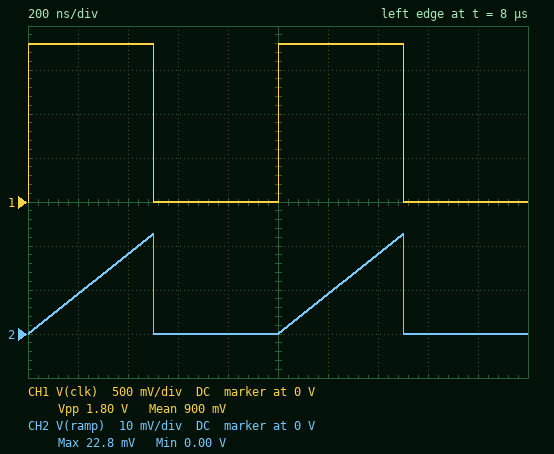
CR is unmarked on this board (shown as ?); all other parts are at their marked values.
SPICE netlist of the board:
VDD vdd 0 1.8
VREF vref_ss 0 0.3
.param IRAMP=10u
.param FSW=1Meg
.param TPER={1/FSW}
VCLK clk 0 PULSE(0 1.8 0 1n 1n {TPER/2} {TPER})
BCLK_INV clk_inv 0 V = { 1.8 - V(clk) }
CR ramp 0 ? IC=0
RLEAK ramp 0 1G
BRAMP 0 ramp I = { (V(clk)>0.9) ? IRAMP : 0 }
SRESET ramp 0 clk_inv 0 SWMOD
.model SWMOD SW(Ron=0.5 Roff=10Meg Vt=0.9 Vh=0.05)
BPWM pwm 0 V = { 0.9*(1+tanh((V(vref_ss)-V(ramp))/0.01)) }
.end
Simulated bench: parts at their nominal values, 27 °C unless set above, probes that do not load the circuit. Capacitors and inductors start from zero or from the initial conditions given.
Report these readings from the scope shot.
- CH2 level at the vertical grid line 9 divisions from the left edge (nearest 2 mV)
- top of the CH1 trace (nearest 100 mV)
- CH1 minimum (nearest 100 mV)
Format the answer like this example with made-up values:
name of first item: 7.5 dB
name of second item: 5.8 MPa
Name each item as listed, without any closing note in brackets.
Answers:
CH2 level at the vertical grid line 9 divisions from the left edge: 0 V
top of the CH1 trace: 1.8 V
CH1 minimum: 0 V
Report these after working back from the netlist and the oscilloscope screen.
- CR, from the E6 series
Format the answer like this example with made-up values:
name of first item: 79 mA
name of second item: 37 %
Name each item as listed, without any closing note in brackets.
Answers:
CR, from the E6 series: 220 pF
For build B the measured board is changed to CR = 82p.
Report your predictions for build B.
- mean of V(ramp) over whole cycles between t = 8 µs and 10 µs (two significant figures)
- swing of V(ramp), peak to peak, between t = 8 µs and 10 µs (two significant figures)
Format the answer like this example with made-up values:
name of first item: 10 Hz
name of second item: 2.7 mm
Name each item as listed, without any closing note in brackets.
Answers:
mean of V(ramp) over whole cycles between t = 8 µs and 10 µs: 15 mV
swing of V(ramp), peak to peak, between t = 8 µs and 10 µs: 61 mV
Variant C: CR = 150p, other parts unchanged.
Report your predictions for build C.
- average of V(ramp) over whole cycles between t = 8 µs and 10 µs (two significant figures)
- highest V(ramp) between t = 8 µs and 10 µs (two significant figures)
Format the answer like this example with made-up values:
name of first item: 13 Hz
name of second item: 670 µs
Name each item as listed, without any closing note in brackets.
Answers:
average of V(ramp) over whole cycles between t = 8 µs and 10 µs: 8.4 mV
highest V(ramp) between t = 8 µs and 10 µs: 33 mV
